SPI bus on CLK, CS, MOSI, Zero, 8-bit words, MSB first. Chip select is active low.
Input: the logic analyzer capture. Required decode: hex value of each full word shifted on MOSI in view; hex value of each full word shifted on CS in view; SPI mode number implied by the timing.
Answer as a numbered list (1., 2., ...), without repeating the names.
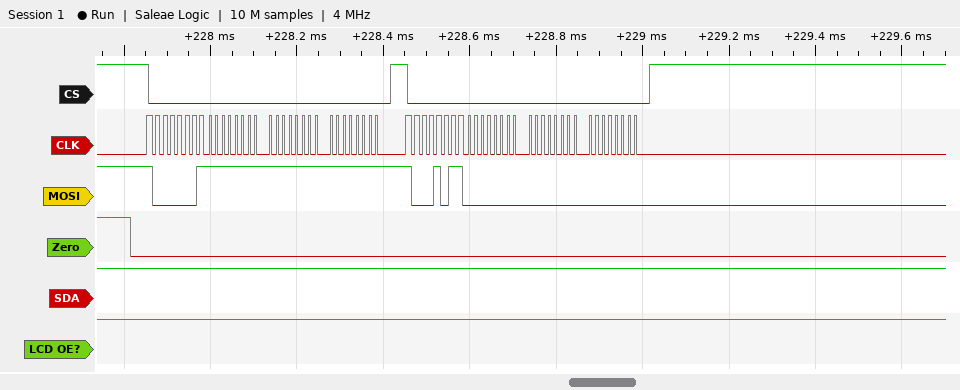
1. 81, FF, FF, FF, 8B, 00, 00, 00
2. 80, 00, 00, 00, 80, 00, 00, 00
3. 0
